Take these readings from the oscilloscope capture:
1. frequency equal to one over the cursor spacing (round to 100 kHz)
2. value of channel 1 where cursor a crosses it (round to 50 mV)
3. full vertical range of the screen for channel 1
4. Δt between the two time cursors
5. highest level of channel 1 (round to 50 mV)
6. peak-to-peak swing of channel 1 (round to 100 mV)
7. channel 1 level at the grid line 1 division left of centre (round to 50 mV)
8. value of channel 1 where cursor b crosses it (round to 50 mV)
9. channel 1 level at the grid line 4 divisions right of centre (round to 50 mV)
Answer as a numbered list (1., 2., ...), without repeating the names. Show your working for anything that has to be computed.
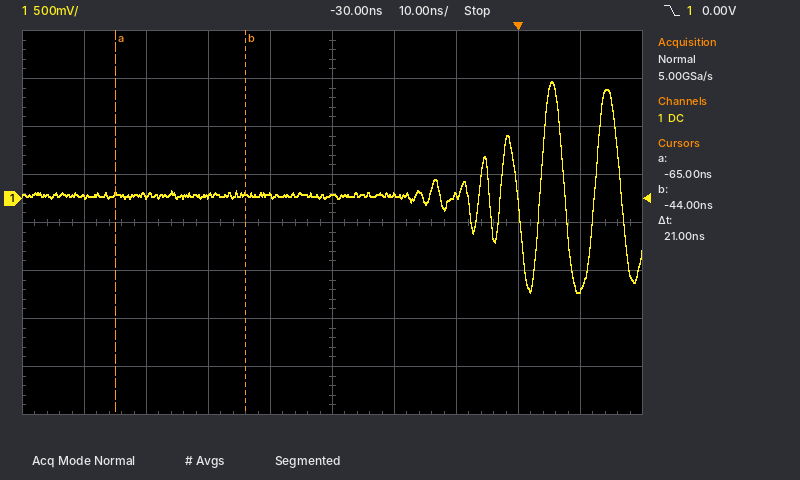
1. 1 / 21 ns ≈ 47.6 MHz
2. 50 mV
3. 4 V
4. 21 ns
5. 1.20 V
6. 2.20 V
7. 50 mV
8. 50 mV
9. -950 mV
